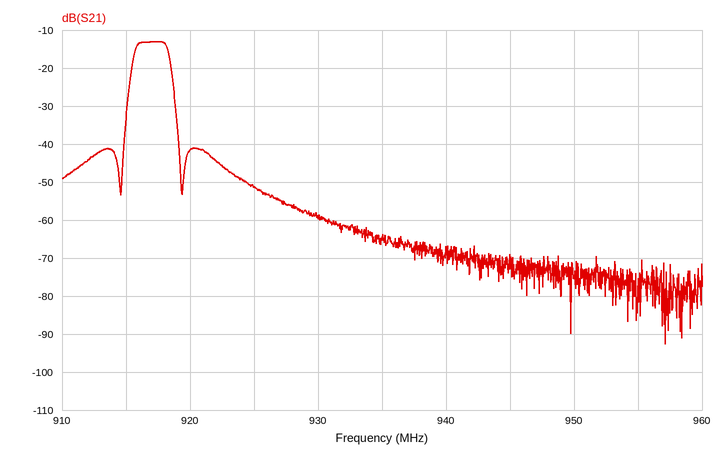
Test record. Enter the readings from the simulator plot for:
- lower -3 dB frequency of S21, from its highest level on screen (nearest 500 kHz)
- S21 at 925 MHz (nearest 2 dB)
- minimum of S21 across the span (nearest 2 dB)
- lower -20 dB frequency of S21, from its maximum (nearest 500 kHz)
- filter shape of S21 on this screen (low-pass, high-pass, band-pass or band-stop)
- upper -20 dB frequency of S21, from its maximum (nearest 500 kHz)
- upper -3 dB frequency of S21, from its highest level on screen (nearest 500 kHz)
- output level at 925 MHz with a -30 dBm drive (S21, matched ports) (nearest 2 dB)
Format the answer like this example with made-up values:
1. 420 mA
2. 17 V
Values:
1. 915.5 MHz
2. -52 dB
3. -92 dB
4. 915.0 MHz
5. band-pass
6. 919.0 MHz
7. 918.5 MHz
8. -82 dBm
